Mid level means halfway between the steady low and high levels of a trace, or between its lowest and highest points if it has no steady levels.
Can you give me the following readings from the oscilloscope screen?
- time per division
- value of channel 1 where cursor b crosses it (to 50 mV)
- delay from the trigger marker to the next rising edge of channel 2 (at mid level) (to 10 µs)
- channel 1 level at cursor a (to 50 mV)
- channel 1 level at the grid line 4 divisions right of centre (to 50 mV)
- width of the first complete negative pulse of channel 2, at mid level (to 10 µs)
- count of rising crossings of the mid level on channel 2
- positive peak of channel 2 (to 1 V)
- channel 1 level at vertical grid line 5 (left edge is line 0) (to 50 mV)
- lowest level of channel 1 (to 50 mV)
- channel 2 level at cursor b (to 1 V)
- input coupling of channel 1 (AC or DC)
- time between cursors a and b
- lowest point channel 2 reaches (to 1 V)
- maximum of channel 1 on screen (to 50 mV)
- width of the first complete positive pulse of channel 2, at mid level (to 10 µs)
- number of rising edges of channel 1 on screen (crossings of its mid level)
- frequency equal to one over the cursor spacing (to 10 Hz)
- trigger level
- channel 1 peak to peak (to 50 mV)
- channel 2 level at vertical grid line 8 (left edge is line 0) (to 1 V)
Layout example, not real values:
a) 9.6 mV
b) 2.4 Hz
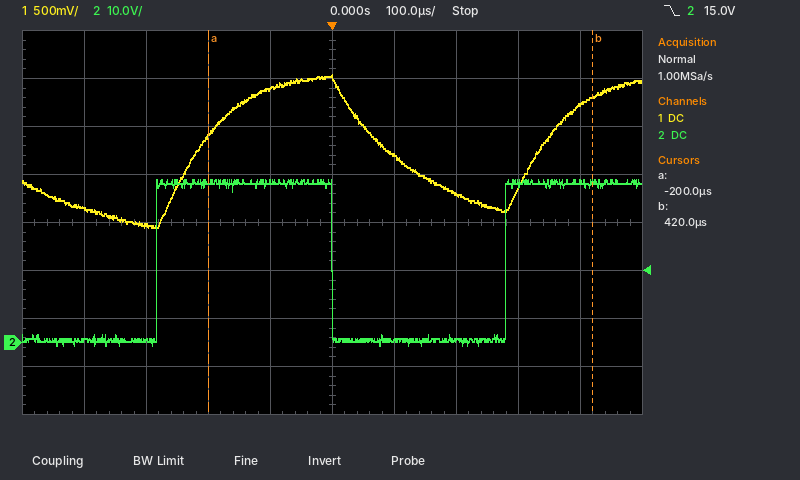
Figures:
a) 100 µs
b) 2.55 V
c) 280 µs
d) 2.15 V
e) 2.50 V
f) 280 µs
g) 2
h) 34 V
i) 2.75 V
j) 1.20 V
k) 33 V
l) DC
m) 620 µs
n) -1 V
o) 2.80 V
p) 280 µs
q) 2
r) 1.61 kHz
s) 15.0 V
t) 1.60 V
u) 33 V
